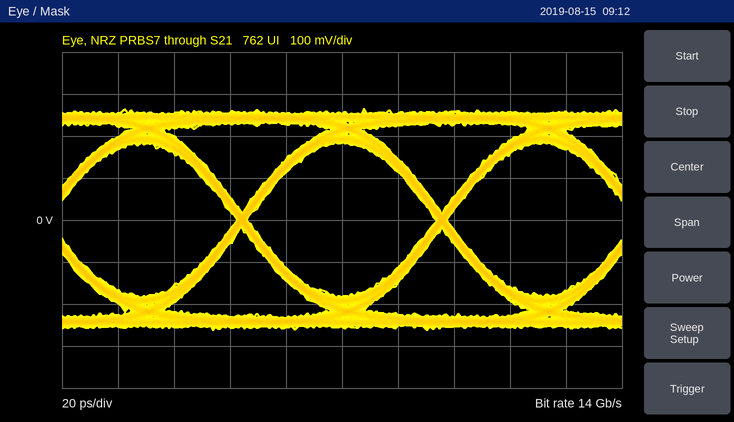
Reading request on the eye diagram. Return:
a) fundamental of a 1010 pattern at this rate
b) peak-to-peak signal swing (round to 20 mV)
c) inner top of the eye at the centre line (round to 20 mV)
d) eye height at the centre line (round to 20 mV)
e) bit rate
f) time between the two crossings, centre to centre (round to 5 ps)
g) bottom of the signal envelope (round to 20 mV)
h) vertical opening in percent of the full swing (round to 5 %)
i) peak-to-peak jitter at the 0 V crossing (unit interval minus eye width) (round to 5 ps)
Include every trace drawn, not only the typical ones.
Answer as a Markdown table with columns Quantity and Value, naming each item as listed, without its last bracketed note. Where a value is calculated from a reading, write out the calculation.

| Quantity | Value |
|---|---|
| fundamental of a 1010 pattern at this rate | 7 GHz |
| peak-to-peak signal swing | 520 mV |
| inner top of the eye at the centre line | 180 mV |
| eye height at the centre line | 360 mV |
| bit rate | 14 Gb/s |
| time between the two crossings, centre to centre | 70 ps |
| bottom of the signal envelope | -260 mV |
| vertical opening in percent of the full swing | 360 mV / 520 mV ≈ 69.2 %, so 70 % to the nearest 5 % |
| peak-to-peak jitter at the 0 V crossing (unit interval minus eye width) | 5 ps |
